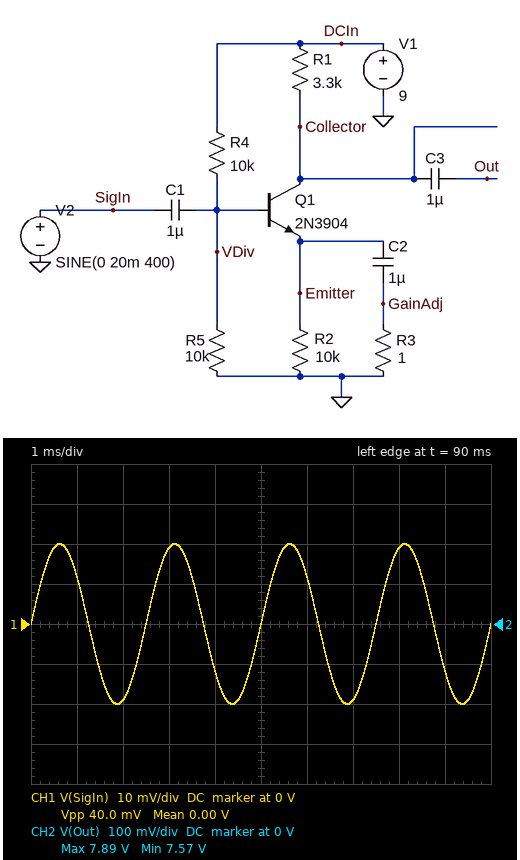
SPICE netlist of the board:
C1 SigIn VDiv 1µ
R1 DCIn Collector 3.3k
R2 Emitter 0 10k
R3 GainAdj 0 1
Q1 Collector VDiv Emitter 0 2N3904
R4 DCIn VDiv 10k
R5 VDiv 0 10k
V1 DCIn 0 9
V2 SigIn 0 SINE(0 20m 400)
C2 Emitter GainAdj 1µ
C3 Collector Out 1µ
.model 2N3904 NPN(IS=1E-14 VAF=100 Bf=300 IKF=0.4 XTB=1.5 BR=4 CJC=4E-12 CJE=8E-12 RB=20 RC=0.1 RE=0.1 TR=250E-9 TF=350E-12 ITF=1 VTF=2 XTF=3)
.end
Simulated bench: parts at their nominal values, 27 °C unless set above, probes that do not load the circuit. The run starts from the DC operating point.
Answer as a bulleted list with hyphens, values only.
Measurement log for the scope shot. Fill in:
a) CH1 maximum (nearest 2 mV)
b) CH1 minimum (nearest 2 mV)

- 20 mV
- -20 mV
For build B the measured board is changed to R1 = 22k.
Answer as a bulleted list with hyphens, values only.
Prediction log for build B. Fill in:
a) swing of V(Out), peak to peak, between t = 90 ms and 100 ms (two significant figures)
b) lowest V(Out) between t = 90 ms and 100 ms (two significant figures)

- 19 mV
- 3.4 V
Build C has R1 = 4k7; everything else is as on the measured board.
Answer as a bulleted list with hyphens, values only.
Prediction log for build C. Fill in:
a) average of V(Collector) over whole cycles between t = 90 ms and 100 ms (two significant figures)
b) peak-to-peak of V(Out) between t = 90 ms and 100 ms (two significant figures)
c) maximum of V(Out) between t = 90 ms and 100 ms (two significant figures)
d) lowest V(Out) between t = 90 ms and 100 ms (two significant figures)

- 7.2 V
- 460 mV
- 7.4 V
- 7.0 V
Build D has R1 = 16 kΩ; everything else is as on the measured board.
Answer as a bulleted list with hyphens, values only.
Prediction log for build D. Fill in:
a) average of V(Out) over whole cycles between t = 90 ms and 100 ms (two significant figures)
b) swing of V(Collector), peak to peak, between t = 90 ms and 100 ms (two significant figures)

- 3.7 V
- 32 mV
